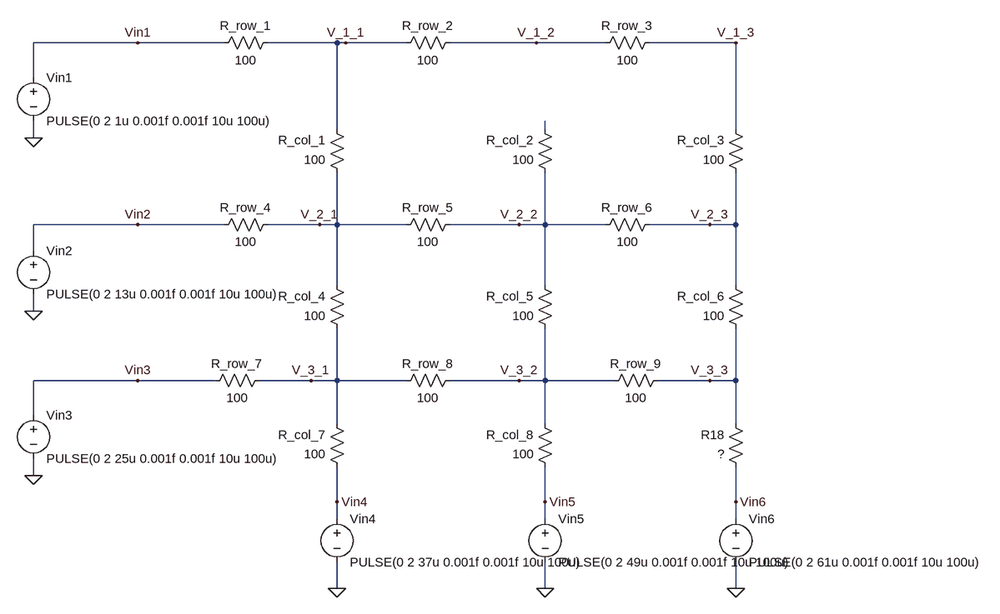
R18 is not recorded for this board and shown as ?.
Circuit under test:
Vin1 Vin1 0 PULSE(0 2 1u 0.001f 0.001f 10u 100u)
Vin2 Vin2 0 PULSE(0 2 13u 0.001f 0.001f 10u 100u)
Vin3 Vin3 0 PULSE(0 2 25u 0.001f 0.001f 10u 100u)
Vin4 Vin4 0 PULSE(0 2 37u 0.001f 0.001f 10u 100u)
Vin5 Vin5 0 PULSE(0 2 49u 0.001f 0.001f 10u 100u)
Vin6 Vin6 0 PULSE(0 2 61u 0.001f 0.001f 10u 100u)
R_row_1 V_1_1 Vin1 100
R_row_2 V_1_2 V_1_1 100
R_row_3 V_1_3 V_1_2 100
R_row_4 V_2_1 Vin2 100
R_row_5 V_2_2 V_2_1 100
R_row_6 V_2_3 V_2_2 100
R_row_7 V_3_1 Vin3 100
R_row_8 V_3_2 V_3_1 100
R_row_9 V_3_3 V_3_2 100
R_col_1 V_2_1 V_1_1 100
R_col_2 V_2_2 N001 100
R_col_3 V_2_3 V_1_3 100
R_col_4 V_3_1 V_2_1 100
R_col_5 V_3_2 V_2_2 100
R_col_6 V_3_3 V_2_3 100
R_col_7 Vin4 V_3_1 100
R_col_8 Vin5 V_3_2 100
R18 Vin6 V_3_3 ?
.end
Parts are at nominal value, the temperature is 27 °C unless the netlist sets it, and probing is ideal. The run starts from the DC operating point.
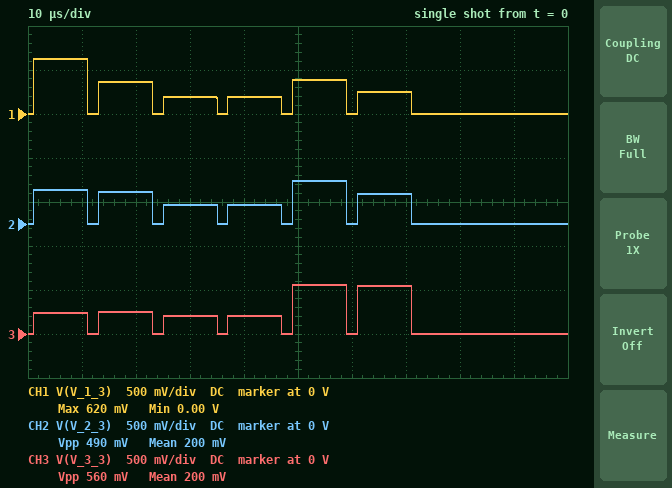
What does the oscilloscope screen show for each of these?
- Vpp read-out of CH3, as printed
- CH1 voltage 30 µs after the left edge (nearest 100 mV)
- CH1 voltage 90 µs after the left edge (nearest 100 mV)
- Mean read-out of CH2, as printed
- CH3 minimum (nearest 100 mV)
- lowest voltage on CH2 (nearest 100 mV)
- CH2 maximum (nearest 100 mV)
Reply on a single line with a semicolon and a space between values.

560 mV; 200 mV; 0 V; 200 mV; 0 V; 0 V; 500 mV
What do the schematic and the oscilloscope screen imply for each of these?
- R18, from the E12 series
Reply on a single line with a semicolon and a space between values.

270 Ω
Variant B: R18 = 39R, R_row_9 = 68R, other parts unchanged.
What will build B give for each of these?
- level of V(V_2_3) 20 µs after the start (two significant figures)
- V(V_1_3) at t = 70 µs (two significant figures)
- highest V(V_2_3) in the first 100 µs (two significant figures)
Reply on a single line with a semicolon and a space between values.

260 mV; 670 mV; 880 mV
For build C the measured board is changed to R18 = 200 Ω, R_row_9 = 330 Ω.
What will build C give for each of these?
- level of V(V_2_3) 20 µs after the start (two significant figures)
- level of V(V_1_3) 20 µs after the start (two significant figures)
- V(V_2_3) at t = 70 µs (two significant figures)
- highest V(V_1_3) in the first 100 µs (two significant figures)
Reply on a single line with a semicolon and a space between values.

350 mV; 360 mV; 500 mV; 620 mV
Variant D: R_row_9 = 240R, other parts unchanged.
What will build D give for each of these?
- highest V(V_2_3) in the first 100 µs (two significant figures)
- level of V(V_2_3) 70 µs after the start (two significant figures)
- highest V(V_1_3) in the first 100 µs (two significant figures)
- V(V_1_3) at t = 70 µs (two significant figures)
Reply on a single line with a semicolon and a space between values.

440 mV; 400 mV; 630 mV; 300 mV
